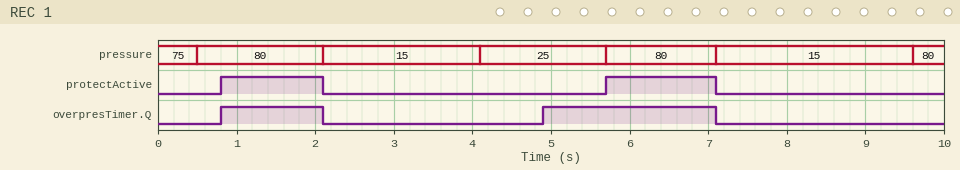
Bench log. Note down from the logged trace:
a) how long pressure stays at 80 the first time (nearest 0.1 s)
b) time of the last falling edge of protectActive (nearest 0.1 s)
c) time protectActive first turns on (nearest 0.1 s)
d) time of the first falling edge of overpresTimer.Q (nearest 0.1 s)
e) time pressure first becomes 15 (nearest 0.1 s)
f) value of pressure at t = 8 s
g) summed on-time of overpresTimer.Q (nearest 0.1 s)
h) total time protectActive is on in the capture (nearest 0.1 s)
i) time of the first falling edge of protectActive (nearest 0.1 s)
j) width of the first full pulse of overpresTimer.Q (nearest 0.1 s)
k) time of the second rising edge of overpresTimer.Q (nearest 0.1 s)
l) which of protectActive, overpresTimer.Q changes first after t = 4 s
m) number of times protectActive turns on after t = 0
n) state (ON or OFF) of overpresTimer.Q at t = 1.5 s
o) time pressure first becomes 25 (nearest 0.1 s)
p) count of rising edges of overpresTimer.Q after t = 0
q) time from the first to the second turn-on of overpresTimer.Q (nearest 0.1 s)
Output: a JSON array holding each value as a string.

["1.6 s", "7.1 s", "0.8 s", "2.1 s", "2.1 s", "15", "3.5 s", "2.7 s", "2.1 s", "1.3 s", "4.9 s", "overpresTimer.Q", "2", "ON", "4.1 s", "2", "4.1 s"]
